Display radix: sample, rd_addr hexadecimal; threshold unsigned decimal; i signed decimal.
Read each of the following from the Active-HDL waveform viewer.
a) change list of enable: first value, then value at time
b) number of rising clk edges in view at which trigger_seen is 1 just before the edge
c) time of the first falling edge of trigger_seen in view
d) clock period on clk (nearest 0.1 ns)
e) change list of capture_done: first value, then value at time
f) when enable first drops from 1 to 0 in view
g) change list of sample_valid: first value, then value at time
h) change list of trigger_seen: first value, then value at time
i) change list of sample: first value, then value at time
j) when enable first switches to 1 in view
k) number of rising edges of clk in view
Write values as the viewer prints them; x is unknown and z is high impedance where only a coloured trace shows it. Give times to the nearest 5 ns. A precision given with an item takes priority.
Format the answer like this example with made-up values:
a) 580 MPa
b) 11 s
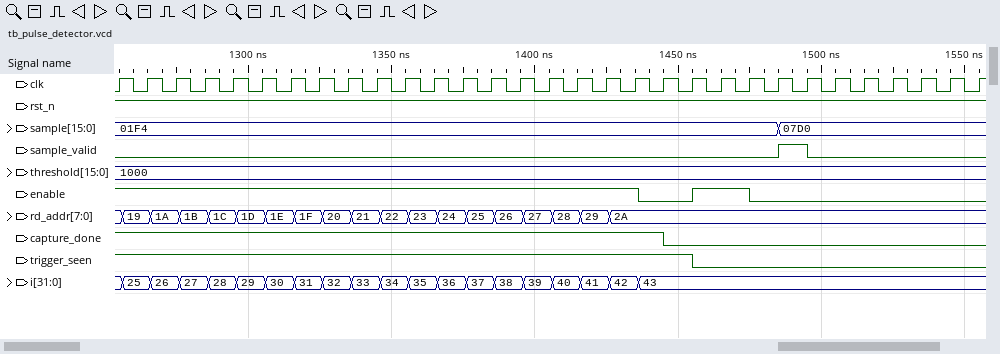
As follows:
a) 1, 0 at 1435 ns, 1 at 1455 ns, 0 at 1475 ns
b) 21
c) 1455 ns
d) 10 ns
e) 1, 0 at 1445 ns
f) 1435 ns
g) 0, 1 at 1485 ns, 0 at 1495 ns
h) 1, 0 at 1455 ns
i) 01F4, 07D0 at 1485 ns
j) 1455 ns
k) 31
